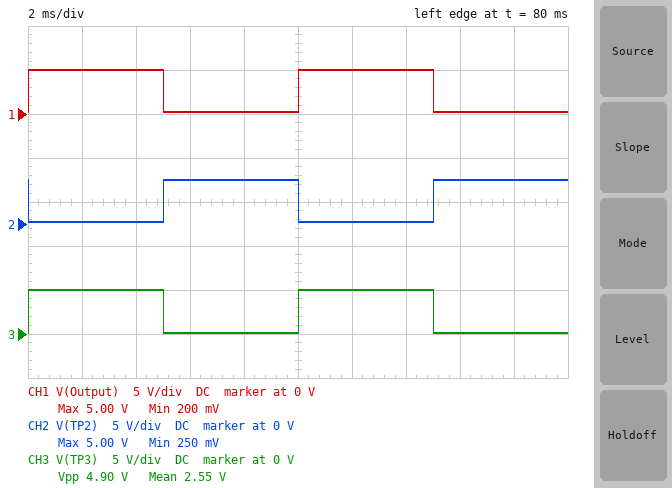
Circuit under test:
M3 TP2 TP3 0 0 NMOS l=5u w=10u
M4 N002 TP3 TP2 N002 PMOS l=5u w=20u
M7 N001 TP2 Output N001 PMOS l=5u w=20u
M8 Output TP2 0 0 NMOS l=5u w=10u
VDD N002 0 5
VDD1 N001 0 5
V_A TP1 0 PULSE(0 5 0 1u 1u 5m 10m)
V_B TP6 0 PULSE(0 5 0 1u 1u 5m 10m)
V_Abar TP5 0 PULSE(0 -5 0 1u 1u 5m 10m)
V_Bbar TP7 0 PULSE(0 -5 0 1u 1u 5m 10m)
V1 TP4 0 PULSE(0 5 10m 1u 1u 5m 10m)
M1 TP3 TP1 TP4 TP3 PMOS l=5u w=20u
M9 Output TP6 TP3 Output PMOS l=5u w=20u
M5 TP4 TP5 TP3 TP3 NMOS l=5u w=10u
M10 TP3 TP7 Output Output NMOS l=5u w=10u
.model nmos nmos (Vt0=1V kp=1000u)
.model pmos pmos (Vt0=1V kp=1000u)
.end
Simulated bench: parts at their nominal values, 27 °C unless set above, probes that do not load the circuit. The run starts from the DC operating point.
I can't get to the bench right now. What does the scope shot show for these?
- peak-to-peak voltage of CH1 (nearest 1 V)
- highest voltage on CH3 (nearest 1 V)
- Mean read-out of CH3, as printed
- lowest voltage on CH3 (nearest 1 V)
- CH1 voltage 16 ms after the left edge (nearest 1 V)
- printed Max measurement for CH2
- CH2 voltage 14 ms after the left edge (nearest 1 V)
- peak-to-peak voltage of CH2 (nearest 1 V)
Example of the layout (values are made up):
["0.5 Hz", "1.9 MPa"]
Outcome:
["5 V", "5 V", "2.55 V", "0 V", "0 V", "5.00 V", "0 V", "5 V"]
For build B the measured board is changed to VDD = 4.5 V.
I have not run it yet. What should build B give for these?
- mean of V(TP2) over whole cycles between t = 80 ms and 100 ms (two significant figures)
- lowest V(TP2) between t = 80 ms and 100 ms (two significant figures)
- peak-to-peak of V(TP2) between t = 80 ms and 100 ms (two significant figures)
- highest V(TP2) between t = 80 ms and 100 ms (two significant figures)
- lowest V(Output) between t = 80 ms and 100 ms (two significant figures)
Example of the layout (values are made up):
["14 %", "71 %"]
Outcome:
["2.3 V", "63 mV", "4.4 V", "4.5 V", "500 mV"]
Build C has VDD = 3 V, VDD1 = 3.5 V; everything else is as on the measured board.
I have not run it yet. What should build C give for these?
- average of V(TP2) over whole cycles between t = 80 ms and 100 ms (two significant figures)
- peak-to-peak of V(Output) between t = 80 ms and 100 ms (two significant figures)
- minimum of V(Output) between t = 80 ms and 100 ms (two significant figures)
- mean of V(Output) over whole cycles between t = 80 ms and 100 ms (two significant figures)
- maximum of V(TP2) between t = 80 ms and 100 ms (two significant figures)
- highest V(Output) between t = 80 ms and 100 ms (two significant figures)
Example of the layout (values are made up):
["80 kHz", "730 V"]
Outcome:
["1.5 V", "2.9 V", "750 mV", "2.2 V", "3.0 V", "3.7 V"]
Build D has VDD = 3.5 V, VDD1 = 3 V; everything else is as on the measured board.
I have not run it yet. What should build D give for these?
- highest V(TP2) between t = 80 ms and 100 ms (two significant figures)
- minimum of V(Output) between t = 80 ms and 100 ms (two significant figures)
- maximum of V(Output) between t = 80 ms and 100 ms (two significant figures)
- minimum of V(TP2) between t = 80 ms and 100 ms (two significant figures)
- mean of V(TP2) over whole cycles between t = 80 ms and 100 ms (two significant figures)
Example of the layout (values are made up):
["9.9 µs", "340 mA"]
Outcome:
["3.5 V", "71 mV", "3.6 V", "13 mV", "1.8 V"]
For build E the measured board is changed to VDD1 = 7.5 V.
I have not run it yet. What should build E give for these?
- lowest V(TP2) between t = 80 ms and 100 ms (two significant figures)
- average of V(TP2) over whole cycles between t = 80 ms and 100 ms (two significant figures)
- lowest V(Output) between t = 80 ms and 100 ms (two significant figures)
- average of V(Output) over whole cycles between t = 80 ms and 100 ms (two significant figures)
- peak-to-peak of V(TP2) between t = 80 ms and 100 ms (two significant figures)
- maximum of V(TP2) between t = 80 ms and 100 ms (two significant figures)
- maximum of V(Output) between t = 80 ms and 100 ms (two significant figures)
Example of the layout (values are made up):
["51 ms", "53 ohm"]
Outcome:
["14 mV", "2.5 V", "1.4 V", "4.0 V", "5.0 V", "5.0 V", "6.5 V"]
